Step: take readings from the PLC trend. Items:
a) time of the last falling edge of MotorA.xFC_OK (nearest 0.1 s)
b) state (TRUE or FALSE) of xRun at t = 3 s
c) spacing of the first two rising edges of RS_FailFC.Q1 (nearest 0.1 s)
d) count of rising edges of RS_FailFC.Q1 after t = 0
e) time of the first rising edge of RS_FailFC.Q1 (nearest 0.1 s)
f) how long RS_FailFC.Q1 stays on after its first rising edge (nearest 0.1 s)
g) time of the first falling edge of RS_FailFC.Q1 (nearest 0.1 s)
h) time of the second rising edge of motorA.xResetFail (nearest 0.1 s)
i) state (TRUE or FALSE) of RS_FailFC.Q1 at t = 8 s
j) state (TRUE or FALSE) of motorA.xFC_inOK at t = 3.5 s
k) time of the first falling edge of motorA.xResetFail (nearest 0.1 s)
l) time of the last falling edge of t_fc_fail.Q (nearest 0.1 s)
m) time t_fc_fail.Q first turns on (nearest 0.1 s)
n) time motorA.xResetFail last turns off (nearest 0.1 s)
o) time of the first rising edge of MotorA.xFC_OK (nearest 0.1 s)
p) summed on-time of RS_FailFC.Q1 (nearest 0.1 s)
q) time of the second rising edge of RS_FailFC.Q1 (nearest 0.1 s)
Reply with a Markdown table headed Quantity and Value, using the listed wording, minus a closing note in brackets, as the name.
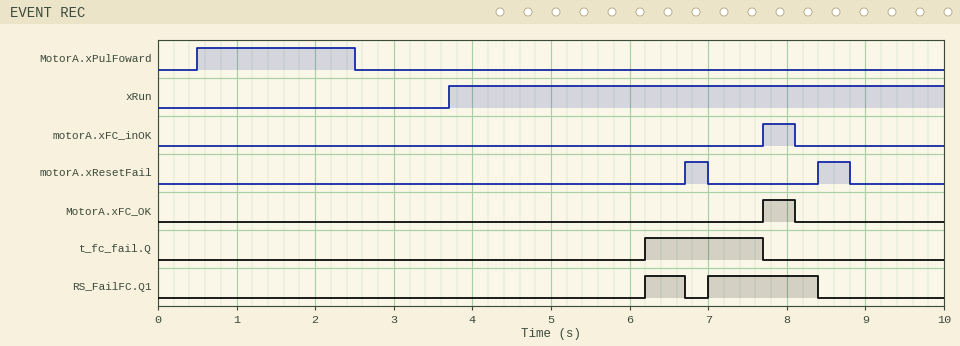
| Quantity | Value |
|---|---|
| time of the last falling edge of MotorA.xFC_OK | 8.1 s |
| state (TRUE or FALSE) of xRun at t = 3 s | FALSE |
| spacing of the first two rising edges of RS_FailFC.Q1 | 0.8 s |
| count of rising edges of RS_FailFC.Q1 after t = 0 | 2 |
| time of the first rising edge of RS_FailFC.Q1 | 6.2 s |
| how long RS_FailFC.Q1 stays on after its first rising edge | 0.5 s |
| time of the first falling edge of RS_FailFC.Q1 | 6.7 s |
| time of the second rising edge of motorA.xResetFail | 8.4 s |
| state (TRUE or FALSE) of RS_FailFC.Q1 at t = 8 s | TRUE |
| state (TRUE or FALSE) of motorA.xFC_inOK at t = 3.5 s | FALSE |
| time of the first falling edge of motorA.xResetFail | 7.0 s |
| time of the last falling edge of t_fc_fail.Q | 7.7 s |
| time t_fc_fail.Q first turns on | 6.2 s |
| time motorA.xResetFail last turns off | 8.8 s |
| time of the first rising edge of MotorA.xFC_OK | 7.7 s |
| summed on-time of RS_FailFC.Q1 | 1.9 s |
| time of the second rising edge of RS_FailFC.Q1 | 7.0 s |
